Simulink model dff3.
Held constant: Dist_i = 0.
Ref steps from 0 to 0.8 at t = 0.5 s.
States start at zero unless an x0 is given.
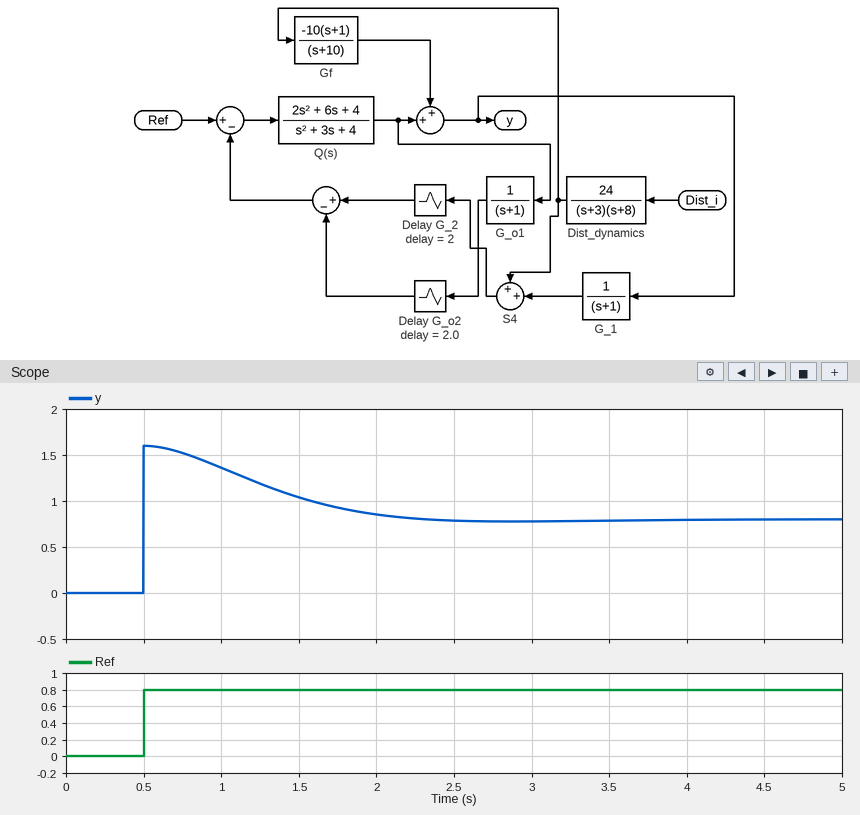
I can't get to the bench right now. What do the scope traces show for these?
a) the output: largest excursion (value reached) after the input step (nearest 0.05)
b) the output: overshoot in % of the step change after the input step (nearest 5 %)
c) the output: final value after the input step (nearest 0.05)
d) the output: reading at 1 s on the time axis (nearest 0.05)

1.60
100 %
0.80
1.35
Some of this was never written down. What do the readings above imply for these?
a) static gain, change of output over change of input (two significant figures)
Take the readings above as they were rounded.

1.0
